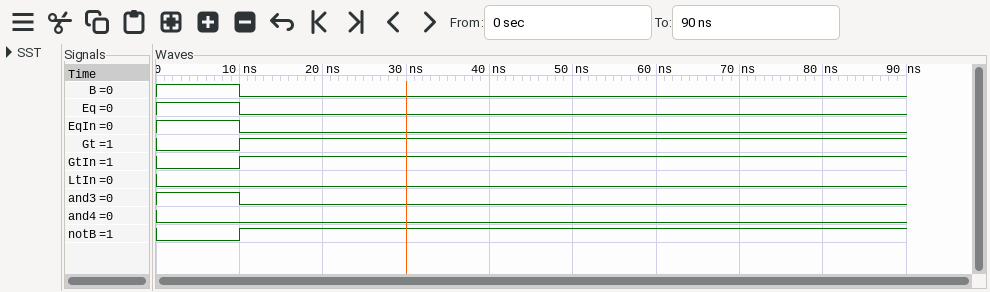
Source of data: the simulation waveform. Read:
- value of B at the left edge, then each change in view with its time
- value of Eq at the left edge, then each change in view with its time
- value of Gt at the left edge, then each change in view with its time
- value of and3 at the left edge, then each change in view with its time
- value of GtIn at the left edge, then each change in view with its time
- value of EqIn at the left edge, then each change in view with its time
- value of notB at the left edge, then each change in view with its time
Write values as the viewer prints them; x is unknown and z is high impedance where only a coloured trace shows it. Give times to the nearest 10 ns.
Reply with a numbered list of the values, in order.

1. 1, 0 at 10 ns
2. 1, 0 at 10 ns
3. 0, 1 at 10 ns
4. 1, 0 at 10 ns
5. 0, 1 at 10 ns
6. 1, 0 at 10 ns
7. 0, 1 at 10 ns
